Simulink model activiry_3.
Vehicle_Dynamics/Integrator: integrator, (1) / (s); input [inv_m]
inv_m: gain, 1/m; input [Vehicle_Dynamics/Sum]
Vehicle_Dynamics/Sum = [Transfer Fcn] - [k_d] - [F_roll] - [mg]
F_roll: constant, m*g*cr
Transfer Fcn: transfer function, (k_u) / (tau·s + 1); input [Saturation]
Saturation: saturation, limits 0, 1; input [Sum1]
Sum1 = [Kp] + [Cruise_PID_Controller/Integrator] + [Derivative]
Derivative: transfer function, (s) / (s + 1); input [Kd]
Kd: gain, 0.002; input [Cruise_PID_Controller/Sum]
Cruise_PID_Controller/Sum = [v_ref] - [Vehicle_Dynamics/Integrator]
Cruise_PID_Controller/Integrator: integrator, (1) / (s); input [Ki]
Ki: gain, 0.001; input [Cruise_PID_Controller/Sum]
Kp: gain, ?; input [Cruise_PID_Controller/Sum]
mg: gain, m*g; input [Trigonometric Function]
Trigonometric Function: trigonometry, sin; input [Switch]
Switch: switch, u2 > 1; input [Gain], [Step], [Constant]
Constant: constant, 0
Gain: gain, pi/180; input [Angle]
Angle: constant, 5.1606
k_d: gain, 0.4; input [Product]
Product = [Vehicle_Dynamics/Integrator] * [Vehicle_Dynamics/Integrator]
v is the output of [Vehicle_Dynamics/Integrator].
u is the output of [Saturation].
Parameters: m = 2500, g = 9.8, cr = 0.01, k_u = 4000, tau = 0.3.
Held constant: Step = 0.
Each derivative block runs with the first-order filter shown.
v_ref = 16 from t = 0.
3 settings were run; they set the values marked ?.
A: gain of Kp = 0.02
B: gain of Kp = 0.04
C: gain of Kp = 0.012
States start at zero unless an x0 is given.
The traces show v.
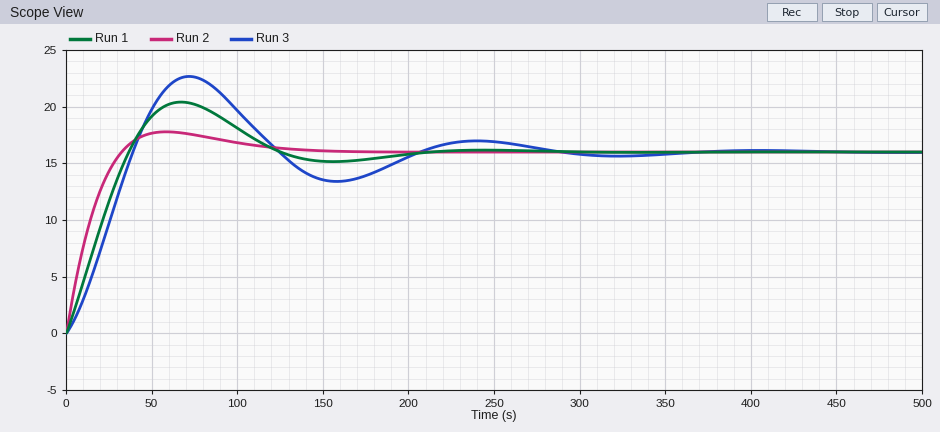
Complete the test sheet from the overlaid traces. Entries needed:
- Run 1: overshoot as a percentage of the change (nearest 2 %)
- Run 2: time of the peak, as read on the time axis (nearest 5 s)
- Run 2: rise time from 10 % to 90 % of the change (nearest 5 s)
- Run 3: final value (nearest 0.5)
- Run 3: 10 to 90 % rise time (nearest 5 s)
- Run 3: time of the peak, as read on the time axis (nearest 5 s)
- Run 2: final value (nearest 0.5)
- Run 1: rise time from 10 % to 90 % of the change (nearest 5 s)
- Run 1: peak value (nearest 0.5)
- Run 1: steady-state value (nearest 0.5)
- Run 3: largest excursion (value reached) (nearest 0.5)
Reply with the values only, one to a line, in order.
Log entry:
28 %
60 s
25 s
16.0
30 s
70 s
16.0
30 s
20.5
16.0
22.5
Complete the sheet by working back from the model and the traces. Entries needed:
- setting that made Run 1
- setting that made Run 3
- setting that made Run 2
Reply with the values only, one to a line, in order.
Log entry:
A
C
B
